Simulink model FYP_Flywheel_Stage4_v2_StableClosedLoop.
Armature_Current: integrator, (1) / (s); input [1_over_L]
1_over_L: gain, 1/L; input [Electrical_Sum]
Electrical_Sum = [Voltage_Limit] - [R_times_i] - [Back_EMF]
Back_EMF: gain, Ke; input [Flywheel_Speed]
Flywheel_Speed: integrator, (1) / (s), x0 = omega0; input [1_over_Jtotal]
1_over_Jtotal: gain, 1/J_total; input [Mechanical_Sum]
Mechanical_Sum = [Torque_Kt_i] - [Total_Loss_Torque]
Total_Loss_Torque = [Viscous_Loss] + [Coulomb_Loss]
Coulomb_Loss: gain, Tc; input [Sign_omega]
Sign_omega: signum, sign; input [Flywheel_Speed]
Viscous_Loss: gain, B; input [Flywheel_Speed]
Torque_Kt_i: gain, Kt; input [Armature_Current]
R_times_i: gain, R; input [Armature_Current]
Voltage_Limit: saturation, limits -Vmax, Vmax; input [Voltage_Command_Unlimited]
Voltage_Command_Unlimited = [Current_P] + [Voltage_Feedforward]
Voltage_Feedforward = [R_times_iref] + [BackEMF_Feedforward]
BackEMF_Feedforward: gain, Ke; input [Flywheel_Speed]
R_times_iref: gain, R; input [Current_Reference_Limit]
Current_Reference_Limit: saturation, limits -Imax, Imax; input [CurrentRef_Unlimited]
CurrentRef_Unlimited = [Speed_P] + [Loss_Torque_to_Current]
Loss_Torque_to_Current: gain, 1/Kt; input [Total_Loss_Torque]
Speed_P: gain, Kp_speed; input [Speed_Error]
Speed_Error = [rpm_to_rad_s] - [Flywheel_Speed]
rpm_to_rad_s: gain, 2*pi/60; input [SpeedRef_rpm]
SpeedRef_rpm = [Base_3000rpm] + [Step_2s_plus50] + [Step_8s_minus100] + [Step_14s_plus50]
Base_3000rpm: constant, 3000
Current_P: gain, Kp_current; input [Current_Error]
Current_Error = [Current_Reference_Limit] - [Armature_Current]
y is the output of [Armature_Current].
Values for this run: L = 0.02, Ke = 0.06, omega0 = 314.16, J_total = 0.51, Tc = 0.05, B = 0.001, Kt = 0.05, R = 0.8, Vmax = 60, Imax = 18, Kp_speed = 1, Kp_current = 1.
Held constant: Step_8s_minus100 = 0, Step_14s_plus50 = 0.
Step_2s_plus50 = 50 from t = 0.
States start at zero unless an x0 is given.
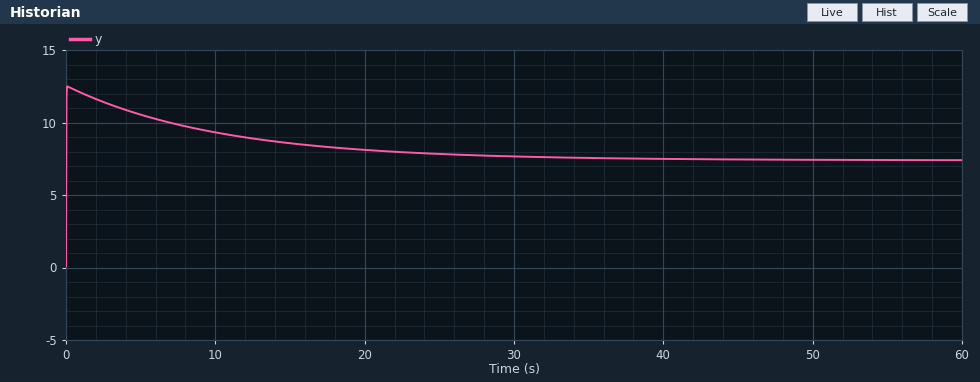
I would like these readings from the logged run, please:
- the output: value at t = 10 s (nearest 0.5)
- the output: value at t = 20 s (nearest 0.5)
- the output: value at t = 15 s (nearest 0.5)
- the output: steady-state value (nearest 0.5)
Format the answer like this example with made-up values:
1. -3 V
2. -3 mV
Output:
1. 9.5
2. 8.0
3. 8.5
4. 7.5
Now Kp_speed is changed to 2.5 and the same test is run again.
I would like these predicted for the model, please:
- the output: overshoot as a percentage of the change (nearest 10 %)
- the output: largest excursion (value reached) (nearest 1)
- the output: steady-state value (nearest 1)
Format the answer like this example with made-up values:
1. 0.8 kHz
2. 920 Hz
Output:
1. 140 %
2. 18
3. 7
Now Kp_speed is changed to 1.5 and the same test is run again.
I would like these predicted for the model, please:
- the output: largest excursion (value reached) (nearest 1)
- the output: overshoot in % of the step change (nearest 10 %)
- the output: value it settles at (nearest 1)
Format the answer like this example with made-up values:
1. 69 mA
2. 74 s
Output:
1. 15
2. 100 %
3. 7
